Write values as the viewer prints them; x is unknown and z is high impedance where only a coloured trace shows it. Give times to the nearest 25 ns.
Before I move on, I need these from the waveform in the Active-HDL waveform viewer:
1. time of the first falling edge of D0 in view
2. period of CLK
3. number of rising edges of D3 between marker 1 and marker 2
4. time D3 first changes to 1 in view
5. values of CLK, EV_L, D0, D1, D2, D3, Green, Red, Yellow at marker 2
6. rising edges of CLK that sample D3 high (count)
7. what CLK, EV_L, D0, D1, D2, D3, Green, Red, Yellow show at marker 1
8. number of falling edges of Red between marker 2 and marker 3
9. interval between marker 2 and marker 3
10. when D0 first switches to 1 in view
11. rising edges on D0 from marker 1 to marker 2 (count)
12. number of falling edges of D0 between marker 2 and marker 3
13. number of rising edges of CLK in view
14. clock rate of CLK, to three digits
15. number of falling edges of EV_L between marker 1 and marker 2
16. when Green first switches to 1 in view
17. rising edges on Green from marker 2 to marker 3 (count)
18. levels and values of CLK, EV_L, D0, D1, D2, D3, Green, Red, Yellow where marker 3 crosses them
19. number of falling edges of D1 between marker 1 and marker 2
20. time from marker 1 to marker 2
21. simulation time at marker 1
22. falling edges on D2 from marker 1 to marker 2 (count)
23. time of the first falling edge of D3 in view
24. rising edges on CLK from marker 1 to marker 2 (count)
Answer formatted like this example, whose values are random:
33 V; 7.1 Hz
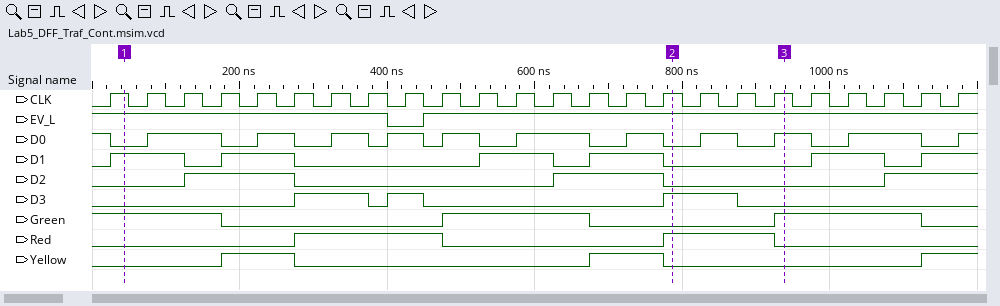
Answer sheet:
25 ns; 50 ns; 3; 275 ns; CLK=1, EV_L=1, D0=0, D1=0, D2=0, D3=1, Green=0, Red=1, Yellow=0; 5; CLK=1, EV_L=1, D0=0, D1=1, D2=0, D3=0, Green=1, Red=0, Yellow=0; 1; 150 ns; 75 ns; 7; 1; 24; 20.0 MHz; 1; 475 ns; 1; CLK=1, EV_L=1, D0=1, D1=0, D2=0, D3=0, Green=1, Red=0, Yellow=0; 4; 750 ns; 50 ns; 2; 375 ns; 15
